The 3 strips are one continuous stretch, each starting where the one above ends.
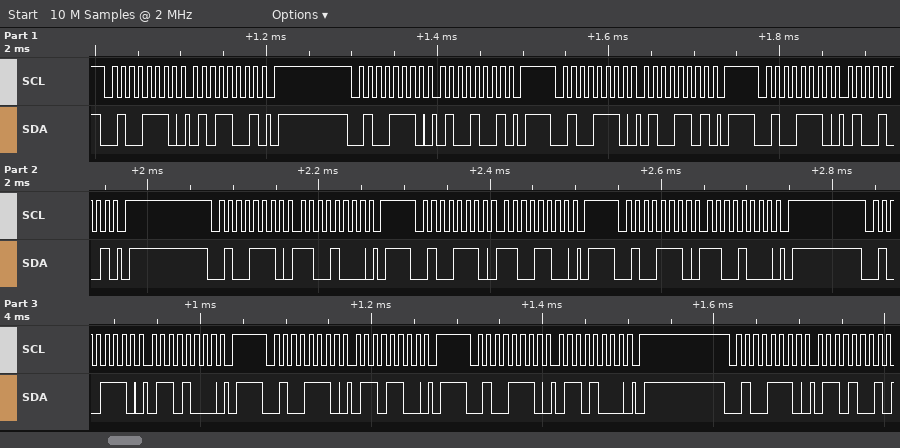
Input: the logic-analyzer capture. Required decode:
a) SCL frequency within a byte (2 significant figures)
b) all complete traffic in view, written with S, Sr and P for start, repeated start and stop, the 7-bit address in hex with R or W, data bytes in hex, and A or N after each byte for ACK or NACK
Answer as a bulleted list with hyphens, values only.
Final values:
- 100 kHz
- S 27W A 59 A P S 27W A 49 A P S 27W A 4D A P S 27W A 49 A P S 27W A C8 A P S 27W A CC A P S 27W A C8 A P S 27W A 68 A P S 27W A 6C A P S 27W A 68 A P S 27W A 69 A
